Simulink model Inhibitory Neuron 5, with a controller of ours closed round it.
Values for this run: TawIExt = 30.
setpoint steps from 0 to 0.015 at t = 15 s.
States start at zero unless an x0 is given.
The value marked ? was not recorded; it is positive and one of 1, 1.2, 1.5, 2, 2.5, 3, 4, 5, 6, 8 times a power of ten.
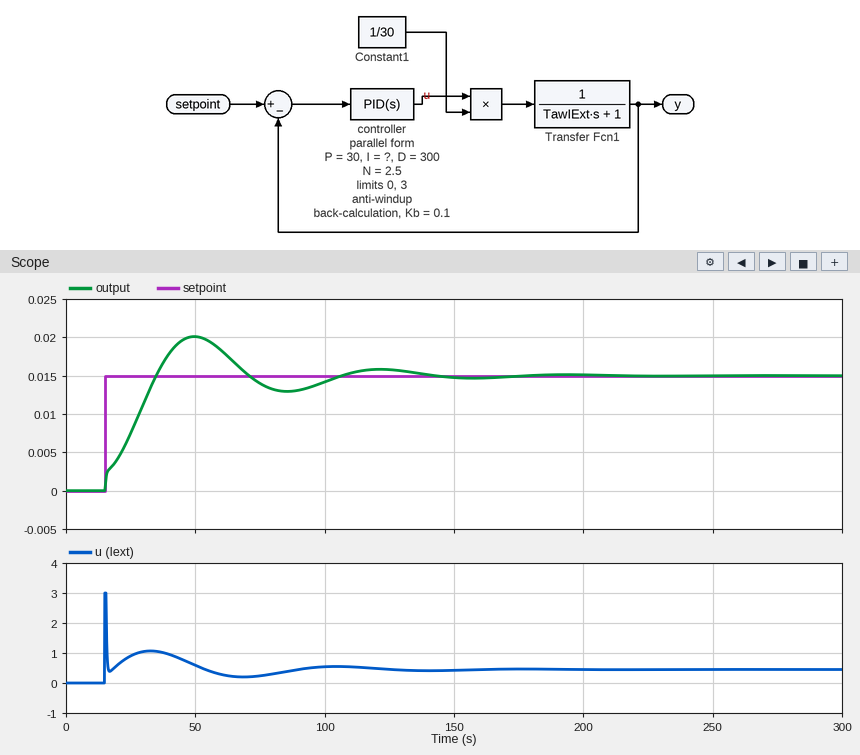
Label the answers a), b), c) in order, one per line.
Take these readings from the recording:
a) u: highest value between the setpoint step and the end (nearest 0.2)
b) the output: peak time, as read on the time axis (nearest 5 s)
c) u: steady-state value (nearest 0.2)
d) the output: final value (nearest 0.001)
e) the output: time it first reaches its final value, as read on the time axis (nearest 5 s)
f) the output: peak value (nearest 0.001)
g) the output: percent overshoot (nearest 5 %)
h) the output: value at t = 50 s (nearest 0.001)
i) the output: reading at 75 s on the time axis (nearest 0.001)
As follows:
a) 3.0
b) 50 s
c) 0.4
d) 0.015
e) 35 s
f) 0.020
g) 35 %
h) 0.020
i) 0.014
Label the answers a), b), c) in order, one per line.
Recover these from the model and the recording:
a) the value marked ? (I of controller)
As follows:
a) 10
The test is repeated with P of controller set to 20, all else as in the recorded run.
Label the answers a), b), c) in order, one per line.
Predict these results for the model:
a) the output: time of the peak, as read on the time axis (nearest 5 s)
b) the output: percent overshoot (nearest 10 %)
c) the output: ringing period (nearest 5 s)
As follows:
a) 50 s
b) 40 %
c) 70 s
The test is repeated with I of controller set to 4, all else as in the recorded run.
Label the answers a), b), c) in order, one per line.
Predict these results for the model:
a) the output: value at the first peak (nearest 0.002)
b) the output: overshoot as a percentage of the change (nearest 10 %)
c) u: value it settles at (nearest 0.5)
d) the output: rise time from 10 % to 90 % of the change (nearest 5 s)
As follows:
a) 0.018
b) 20 %
c) 0.5
d) 30 s
